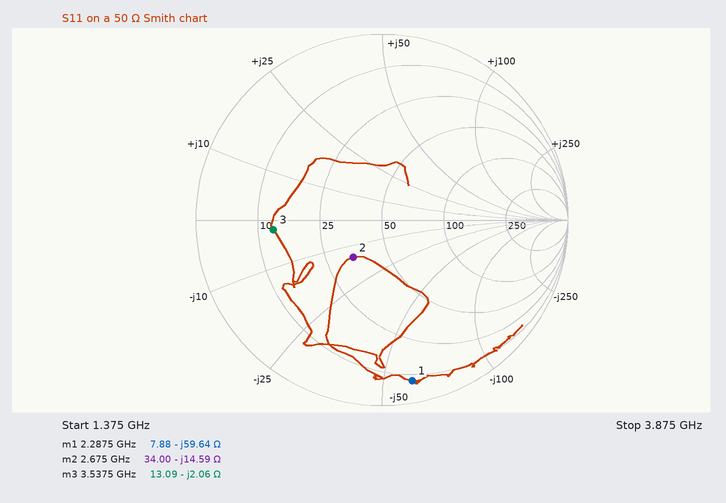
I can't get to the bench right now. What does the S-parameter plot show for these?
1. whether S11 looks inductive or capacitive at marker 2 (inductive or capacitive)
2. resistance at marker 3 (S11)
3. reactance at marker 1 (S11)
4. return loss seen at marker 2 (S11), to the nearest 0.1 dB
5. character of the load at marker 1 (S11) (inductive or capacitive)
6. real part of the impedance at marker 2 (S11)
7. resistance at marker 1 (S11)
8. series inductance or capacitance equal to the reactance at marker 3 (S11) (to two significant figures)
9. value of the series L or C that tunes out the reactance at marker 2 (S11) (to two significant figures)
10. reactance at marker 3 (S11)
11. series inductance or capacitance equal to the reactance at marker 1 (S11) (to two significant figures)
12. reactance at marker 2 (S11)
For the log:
capacitive
13.09 Ω
-59.64 Ω
11.9 dB
capacitive
34.00 Ω
7.88 Ω
22 pF
870 pH
-2.06 Ω
1.2 pF
-14.59 Ω
